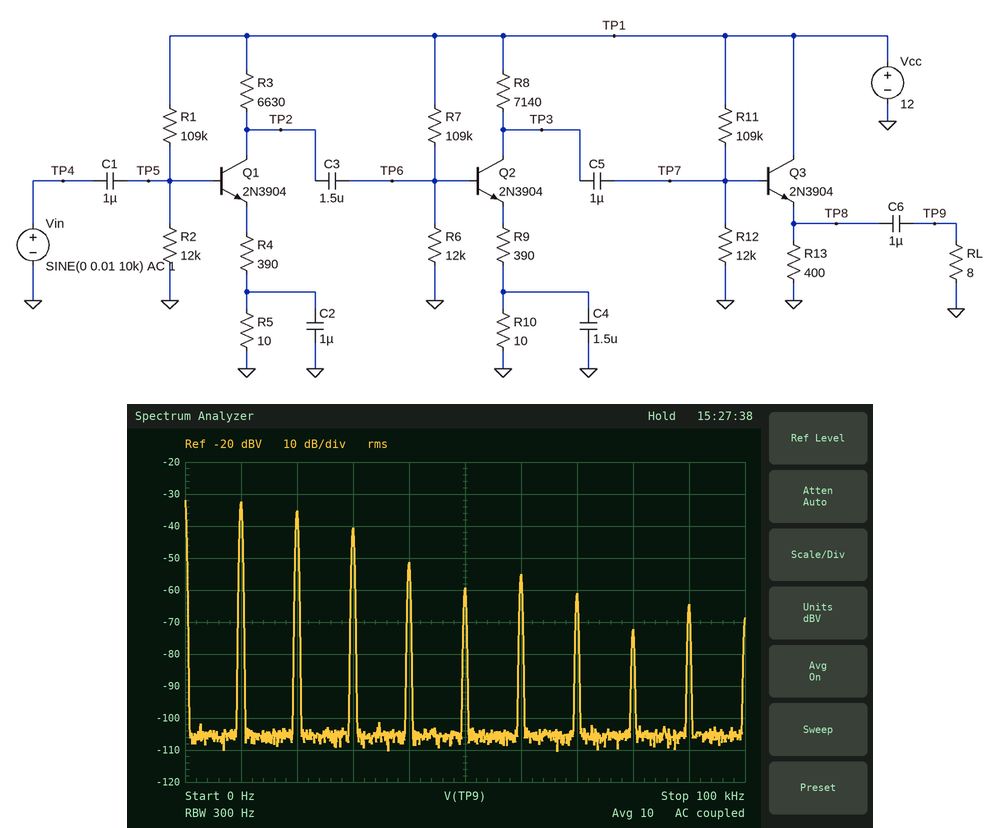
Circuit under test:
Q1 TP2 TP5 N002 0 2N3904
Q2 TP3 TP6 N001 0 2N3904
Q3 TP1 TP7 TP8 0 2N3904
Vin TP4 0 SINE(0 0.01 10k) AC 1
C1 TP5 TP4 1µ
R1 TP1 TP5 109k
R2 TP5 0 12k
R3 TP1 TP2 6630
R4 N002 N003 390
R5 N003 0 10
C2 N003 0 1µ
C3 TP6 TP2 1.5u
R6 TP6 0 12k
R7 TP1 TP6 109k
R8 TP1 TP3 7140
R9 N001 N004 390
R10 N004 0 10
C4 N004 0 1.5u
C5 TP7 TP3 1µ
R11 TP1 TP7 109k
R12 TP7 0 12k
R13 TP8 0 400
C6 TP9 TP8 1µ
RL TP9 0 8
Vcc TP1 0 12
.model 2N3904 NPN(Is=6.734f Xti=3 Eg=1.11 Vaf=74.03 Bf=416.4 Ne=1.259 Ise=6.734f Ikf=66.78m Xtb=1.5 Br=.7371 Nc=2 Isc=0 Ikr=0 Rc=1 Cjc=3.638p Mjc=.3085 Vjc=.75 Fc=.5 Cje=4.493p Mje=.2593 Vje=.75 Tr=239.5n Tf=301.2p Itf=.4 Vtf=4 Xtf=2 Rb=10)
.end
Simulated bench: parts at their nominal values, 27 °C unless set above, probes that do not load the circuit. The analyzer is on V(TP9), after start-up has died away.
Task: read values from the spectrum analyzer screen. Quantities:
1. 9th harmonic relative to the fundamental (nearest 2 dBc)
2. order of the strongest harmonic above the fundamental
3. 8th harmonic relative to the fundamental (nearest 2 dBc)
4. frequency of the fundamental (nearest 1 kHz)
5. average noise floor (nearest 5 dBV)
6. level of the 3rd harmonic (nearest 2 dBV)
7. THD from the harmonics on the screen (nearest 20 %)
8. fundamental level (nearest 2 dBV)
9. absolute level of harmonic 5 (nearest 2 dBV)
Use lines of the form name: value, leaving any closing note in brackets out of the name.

9th harmonic relative to the fundamental: -32 dBc
order of the strongest harmonic above the fundamental: 2
8th harmonic relative to the fundamental: -40 dBc
frequency of the fundamental: 10 kHz
average noise floor: -105 dBV
level of the 3rd harmonic: -40 dBV
THD from the harmonics on the screen: 80 %
fundamental level: -32 dBV
absolute level of harmonic 5: -60 dBV
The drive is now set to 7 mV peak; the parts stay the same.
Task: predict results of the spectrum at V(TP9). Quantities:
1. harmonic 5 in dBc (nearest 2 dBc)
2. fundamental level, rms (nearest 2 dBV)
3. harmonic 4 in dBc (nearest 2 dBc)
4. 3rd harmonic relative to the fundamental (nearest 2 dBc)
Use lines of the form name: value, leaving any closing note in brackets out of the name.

harmonic 5 in dBc: -24 dBc
fundamental level, rms: -34 dBV
harmonic 4 in dBc: -24 dBc
3rd harmonic relative to the fundamental: -10 dBc
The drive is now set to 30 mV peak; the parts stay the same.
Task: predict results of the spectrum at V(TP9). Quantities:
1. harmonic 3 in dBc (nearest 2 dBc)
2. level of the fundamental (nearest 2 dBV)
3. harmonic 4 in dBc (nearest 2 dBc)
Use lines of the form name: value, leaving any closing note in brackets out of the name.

harmonic 3 in dBc: -6 dBc
level of the fundamental: -26 dBV
harmonic 4 in dBc: -14 dBc
